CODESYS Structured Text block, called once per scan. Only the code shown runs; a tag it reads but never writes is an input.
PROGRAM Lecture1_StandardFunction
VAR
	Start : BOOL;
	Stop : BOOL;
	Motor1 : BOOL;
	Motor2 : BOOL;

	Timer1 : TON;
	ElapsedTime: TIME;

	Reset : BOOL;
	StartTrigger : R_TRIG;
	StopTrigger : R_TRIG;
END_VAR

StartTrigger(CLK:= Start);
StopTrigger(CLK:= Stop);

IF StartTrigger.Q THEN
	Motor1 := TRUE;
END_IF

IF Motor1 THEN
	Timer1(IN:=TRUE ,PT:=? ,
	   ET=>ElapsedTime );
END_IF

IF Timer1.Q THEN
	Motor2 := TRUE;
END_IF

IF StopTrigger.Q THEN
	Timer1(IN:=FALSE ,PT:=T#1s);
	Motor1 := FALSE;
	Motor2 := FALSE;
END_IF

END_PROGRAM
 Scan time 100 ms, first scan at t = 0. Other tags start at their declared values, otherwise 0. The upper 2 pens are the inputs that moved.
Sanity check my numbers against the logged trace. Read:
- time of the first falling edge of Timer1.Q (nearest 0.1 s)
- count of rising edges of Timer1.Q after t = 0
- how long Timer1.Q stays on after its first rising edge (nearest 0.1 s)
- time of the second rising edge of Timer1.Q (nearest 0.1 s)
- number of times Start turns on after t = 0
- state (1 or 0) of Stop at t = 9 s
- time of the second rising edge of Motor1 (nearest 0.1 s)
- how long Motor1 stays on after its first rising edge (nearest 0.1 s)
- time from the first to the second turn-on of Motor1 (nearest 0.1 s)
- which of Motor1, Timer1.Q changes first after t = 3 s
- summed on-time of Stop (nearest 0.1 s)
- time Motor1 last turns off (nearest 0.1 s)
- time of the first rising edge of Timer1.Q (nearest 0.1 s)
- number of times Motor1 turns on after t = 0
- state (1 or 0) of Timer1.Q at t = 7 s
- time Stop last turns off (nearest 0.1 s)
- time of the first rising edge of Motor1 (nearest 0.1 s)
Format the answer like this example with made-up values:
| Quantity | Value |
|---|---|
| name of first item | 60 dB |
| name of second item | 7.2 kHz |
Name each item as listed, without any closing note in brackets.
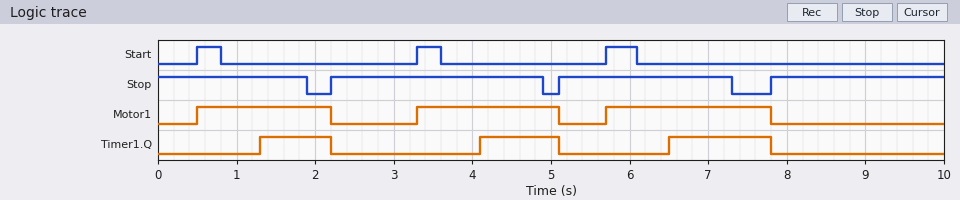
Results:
| Quantity | Value |
|---|---|
| time of the first falling edge of Timer1.Q | 2.2 s |
| count of rising edges of Timer1.Q after t = 0 | 3 |
| how long Timer1.Q stays on after its first rising edge | 0.9 s |
| time of the second rising edge of Timer1.Q | 4.1 s |
| number of times Start turns on after t = 0 | 3 |
| state (1 or 0) of Stop at t = 9 s | 1 |
| time of the second rising edge of Motor1 | 3.3 s |
| how long Motor1 stays on after its first rising edge | 1.7 s |
| time from the first to the second turn-on of Motor1 | 2.8 s |
| which of Motor1, Timer1.Q changes first after t = 3 s | Motor1 |
| summed on-time of Stop | 9.0 s |
| time Motor1 last turns off | 7.8 s |
| time of the first rising edge of Timer1.Q | 1.3 s |
| number of times Motor1 turns on after t = 0 | 3 |
| state (1 or 0) of Timer1.Q at t = 7 s | 1 |
| time Stop last turns off | 7.3 s |
| time of the first rising edge of Motor1 | 0.5 s |
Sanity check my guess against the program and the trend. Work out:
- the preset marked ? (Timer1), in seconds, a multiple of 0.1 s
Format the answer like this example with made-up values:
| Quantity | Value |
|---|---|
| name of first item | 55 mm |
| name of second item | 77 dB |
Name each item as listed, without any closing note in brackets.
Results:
| Quantity | Value |
|---|---|
| the preset marked ? (Timer1), in seconds, a multiple of 0.1 s | 0.8 s |
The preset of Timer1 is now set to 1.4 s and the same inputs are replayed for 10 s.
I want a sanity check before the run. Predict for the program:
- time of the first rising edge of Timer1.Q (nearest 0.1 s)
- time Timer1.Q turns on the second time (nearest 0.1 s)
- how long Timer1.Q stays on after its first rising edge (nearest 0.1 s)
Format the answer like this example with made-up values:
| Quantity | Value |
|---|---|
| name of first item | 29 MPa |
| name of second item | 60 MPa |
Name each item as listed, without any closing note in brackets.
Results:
| Quantity | Value |
|---|---|
| time of the first rising edge of Timer1.Q | 1.9 s |
| time Timer1.Q turns on the second time | 4.7 s |
| how long Timer1.Q stays on after its first rising edge | 0.3 s |
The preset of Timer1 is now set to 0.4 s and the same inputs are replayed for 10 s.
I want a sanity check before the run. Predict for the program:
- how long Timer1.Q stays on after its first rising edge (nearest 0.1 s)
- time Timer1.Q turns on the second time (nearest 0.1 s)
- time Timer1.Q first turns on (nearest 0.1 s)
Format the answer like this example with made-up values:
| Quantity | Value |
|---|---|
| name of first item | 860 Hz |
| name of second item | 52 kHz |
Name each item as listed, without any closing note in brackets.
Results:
| Quantity | Value |
|---|---|
| how long Timer1.Q stays on after its first rising edge | 1.3 s |
| time Timer1.Q turns on the second time | 3.7 s |
| time Timer1.Q first turns on | 0.9 s |
